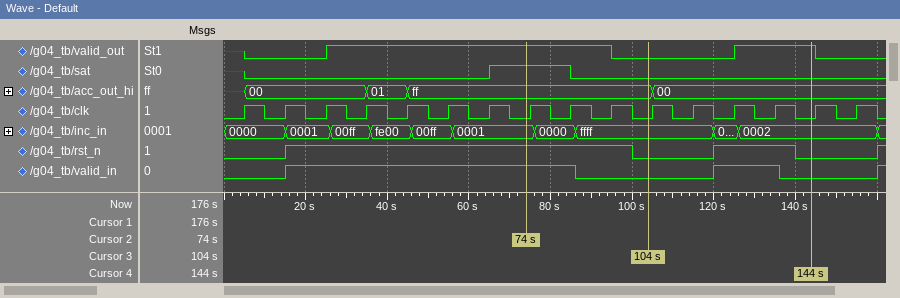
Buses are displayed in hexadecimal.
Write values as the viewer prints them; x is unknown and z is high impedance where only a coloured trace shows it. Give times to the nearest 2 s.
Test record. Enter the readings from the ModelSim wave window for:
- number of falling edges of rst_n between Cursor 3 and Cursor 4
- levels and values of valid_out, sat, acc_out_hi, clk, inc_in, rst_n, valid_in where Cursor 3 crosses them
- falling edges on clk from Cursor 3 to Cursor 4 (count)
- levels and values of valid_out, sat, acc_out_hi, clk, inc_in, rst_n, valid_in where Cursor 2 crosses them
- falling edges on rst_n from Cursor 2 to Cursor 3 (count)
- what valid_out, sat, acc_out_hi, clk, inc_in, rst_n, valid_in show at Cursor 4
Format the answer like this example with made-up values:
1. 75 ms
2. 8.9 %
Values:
1. 1
2. valid_out=0, sat=0, acc_out_hi=ff, clk=0, inc_in=ffff, rst_n=0, valid_in=0
3. 4
4. valid_out=1, sat=1, acc_out_hi=ff, clk=0, inc_in=0001, rst_n=1, valid_in=1
5. 1
6. valid_out=1, sat=0, acc_out_hi=00, clk=0, inc_in=0002, rst_n=0, valid_in=0
